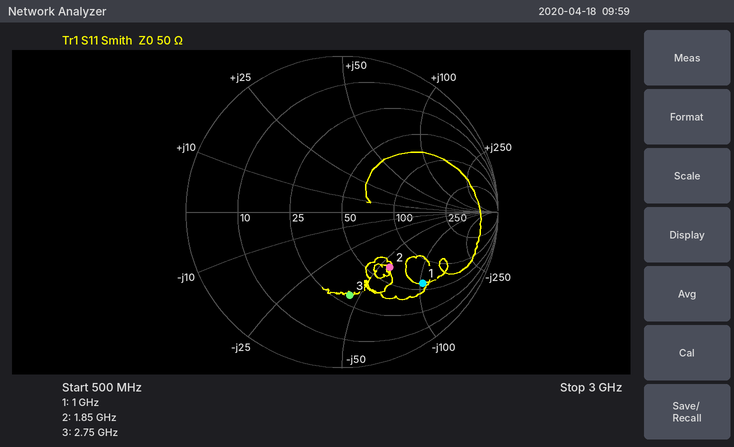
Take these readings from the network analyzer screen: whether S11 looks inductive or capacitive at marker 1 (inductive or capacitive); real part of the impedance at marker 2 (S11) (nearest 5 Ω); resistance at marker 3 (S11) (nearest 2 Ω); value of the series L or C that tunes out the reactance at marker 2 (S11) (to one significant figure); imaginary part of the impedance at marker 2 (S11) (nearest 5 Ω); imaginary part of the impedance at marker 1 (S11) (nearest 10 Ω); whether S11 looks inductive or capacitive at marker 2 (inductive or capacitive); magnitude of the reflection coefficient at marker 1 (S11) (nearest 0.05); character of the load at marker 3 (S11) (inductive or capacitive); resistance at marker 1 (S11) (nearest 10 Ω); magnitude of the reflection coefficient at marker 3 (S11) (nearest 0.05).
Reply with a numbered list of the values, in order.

1. capacitive
2. 65 Ω
3. 30 Ω
4. 5 nH
5. -60 Ω
6. -100 Ω
7. capacitive
8. 0.70
9. capacitive
10. 60 Ω
11. 0.55
